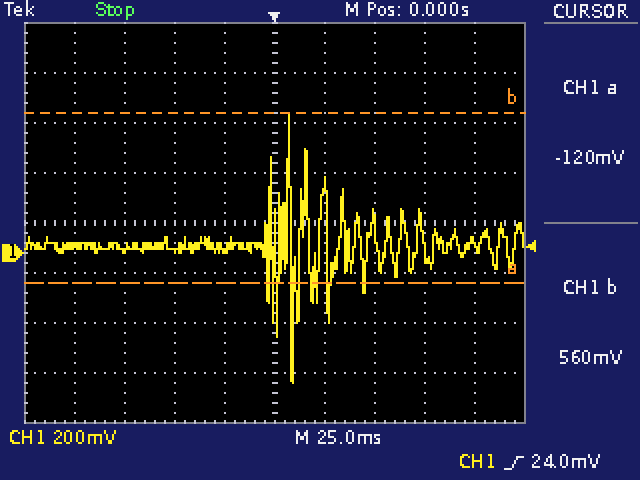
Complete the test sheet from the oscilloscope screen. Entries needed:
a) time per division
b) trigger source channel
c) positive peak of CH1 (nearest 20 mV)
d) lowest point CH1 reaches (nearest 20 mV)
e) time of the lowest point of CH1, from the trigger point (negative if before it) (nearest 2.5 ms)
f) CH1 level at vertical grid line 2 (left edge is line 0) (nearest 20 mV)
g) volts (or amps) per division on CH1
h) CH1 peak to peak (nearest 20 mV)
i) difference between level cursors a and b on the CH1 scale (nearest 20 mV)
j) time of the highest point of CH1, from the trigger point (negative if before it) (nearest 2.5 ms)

25 ms
CH1
560 mV
-520 mV
+10.0 ms
20 mV
200 mV
1.08 V
680 mV
+7.5 ms
